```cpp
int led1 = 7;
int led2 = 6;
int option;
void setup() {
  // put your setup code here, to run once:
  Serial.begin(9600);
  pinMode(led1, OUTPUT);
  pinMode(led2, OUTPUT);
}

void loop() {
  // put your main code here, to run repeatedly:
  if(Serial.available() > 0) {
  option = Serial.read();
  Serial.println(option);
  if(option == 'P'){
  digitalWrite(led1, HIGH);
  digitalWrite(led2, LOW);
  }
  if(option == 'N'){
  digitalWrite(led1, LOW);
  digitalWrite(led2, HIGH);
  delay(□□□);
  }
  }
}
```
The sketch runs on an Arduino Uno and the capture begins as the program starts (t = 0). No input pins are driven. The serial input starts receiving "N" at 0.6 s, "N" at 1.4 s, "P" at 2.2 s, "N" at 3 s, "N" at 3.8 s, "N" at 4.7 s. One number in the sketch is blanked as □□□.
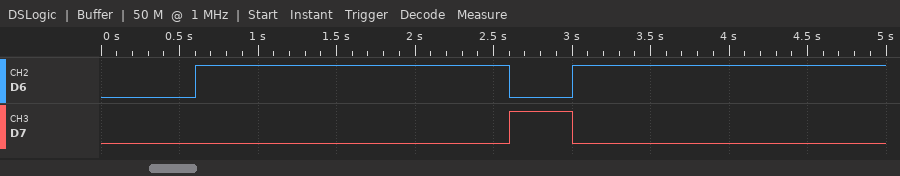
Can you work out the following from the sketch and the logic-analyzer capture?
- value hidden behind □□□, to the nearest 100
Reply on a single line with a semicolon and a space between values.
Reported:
1000
